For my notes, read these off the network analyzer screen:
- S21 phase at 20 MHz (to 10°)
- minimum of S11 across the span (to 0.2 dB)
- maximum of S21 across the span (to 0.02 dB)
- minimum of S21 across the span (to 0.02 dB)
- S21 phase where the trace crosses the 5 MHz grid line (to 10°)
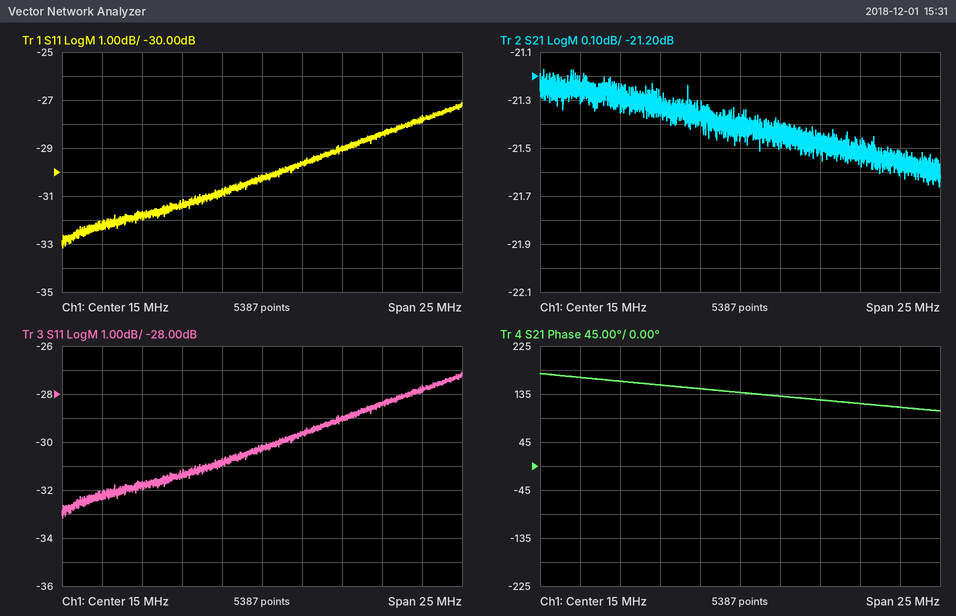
120°
-33.2 dB
-21.18 dB
-21.66 dB
170°
